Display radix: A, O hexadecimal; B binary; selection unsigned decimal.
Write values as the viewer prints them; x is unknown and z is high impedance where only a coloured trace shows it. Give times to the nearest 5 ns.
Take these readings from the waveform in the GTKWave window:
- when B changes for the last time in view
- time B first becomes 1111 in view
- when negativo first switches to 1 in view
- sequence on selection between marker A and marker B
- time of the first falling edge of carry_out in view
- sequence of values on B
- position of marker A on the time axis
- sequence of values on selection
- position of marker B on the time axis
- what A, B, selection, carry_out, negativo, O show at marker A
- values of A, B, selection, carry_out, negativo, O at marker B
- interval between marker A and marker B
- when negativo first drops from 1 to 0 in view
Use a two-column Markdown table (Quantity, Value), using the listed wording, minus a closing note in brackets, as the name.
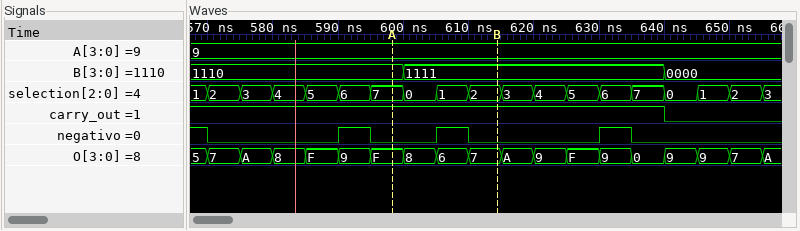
| Quantity | Value |
|---|---|
| when B changes for the last time in view | 640 ns |
| time B first becomes 1111 in view | 600 ns |
| when negativo first switches to 1 in view | 590 ns |
| sequence on selection between marker A and marker B | 7, 0, 1, 2 |
| time of the first falling edge of carry_out in view | 640 ns |
| sequence of values on B | 1110, 1111, 0000 |
| position of marker A on the time axis | 600 ns |
| sequence of values on selection | 1, 2, 3, 4, 5, 6, 7, 0, 1, 2, 3, 4, 5, 6, 7, 0, 1, 2, 3 |
| position of marker B on the time axis | 615 ns |
| what A, B, selection, carry_out, negativo, O show at marker A | A=9, B=1110, selection=7, carry_out=1, negativo=0, O=F |
| values of A, B, selection, carry_out, negativo, O at marker B | A=9, B=1111, selection=2, carry_out=1, negativo=0, O=7 |
| interval between marker A and marker B | 15 ns |
| when negativo first drops from 1 to 0 in view | 570 ns |
